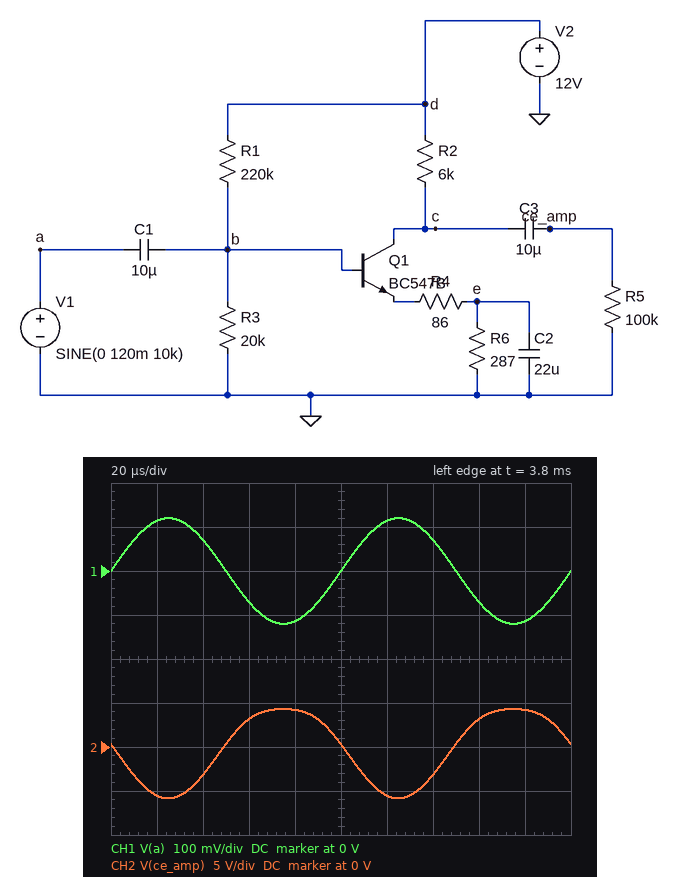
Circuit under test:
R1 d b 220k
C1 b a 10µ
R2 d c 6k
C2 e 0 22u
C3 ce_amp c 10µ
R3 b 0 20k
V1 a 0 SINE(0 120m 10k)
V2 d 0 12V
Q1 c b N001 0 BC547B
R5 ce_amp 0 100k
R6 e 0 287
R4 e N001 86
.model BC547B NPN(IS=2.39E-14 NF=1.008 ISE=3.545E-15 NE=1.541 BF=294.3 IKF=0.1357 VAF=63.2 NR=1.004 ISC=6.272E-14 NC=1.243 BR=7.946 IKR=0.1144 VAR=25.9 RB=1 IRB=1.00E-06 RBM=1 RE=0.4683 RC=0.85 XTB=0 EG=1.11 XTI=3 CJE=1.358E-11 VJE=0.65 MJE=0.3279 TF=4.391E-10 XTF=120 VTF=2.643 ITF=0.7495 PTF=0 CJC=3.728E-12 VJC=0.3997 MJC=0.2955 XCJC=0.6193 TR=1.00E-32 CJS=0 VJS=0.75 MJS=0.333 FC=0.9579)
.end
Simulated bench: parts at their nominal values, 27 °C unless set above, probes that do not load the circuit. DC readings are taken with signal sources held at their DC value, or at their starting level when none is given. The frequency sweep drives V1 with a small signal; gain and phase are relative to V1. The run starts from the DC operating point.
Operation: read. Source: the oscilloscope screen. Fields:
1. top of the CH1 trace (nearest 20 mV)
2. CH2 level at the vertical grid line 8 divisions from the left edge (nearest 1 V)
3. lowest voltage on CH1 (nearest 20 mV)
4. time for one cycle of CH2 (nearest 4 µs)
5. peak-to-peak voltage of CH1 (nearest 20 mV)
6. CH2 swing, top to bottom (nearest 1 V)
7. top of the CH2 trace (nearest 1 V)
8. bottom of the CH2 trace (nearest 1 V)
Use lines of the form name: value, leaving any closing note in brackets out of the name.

top of the CH1 trace: 120 mV
CH2 level at the vertical grid line 8 divisions from the left edge: 3 V
lowest voltage on CH1: -120 mV
time for one cycle of CH2: 100 µs
peak-to-peak voltage of CH1: 240 mV
CH2 swing, top to bottom: 10 V
top of the CH2 trace: 4 V
bottom of the CH2 trace: -6 V
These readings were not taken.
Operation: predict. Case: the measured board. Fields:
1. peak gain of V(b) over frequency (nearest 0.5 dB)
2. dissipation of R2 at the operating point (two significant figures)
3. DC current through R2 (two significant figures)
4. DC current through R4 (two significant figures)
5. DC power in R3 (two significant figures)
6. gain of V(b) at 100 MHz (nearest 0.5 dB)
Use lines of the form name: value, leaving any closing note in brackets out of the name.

peak gain of V(b) over frequency: 0 dB
dissipation of R2 at the operating point: 4.3 mW
DC current through R2: 850 µA
DC current through R4: 850 µA
DC power in R3: 45 µW
gain of V(b) at 100 MHz: 0 dB
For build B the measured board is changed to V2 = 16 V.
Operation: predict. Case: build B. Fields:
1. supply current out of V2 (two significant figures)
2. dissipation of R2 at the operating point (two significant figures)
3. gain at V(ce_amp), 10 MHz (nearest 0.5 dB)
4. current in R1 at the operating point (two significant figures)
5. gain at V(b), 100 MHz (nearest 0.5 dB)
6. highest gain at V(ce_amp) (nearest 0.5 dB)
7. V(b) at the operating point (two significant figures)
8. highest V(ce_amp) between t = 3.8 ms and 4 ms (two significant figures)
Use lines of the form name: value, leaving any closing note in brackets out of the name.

supply current out of V2: 1.6 mA
dissipation of R2 at the operating point: 15 mW
gain at V(ce_amp), 10 MHz: 33.0 dB
current in R1 at the operating point: 67 µA
gain at V(b), 100 MHz: 0 dB
highest gain at V(ce_amp): 34.5 dB
V(b) at the operating point: 1.2 V
highest V(ce_amp) between t = 3.8 ms and 4 ms: 6.0 V
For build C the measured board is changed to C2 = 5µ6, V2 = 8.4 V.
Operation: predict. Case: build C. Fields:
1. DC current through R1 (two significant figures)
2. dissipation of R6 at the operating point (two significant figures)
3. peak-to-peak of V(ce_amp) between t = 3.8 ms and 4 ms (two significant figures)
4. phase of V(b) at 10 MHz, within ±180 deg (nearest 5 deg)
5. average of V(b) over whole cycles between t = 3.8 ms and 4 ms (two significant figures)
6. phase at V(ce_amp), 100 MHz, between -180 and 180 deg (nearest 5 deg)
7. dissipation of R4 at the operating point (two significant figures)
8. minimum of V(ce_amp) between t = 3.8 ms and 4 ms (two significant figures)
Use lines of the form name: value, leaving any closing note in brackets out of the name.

DC current through R1: 35 µA
dissipation of R6 at the operating point: 16 µW
peak-to-peak of V(ce_amp) between t = 3.8 ms and 4 ms: 5.2 V
phase of V(b) at 10 MHz, within ±180 deg: 0 deg
average of V(b) over whole cycles between t = 3.8 ms and 4 ms: 690 mV
phase at V(ce_amp), 100 MHz, between -180 and 180 deg: 45 deg
dissipation of R4 at the operating point: 4.8 µW
minimum of V(ce_amp) between t = 3.8 ms and 4 ms: -3.9 V
